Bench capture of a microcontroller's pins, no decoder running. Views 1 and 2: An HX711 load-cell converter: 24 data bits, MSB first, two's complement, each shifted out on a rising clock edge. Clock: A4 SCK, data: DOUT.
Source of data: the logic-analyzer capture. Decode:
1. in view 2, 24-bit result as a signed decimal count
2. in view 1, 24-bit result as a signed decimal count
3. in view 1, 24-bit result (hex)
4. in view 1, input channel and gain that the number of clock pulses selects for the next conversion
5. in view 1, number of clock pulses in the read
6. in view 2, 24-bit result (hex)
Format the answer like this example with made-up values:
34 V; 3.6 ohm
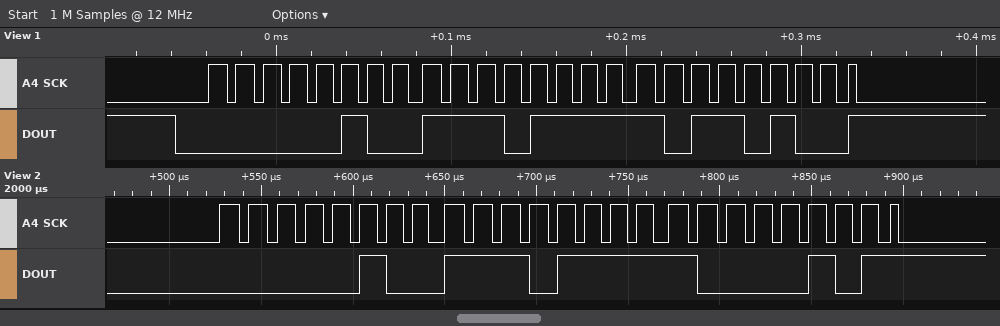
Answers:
323461; 323508; 0x04EFB4; channel A, gain 128; 25; 0x04EF85
